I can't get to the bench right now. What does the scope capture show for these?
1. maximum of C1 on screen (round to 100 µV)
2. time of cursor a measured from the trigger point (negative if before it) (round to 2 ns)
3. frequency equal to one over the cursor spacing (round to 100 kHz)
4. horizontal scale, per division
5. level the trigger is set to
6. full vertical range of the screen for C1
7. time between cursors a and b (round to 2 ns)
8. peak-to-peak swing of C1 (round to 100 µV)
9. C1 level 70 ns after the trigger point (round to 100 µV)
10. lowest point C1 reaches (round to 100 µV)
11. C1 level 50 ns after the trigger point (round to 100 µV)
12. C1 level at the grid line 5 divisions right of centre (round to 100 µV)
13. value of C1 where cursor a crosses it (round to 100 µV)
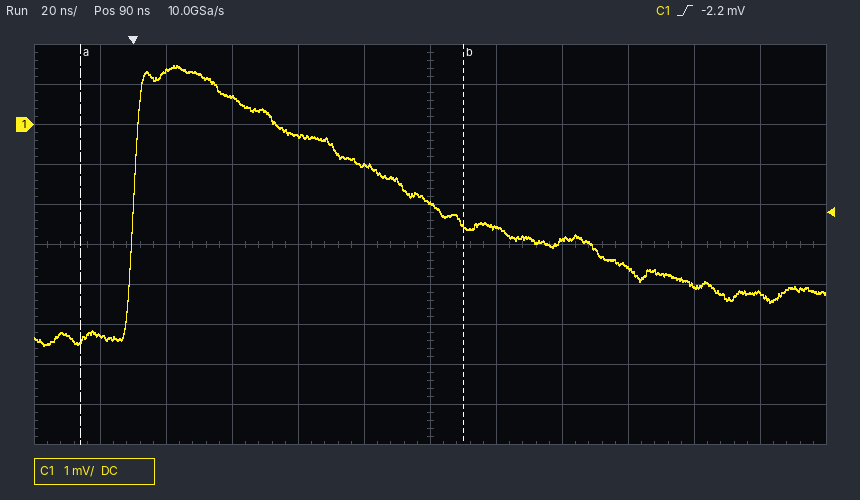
1.5 mV
-16 ns
8.6 MHz
20 ns
-2.2 mV
10 mV
116 ns
7.0 mV
-1.0 mV
-5.5 mV
-300 µV
-4.2 mV
-5.4 mV
